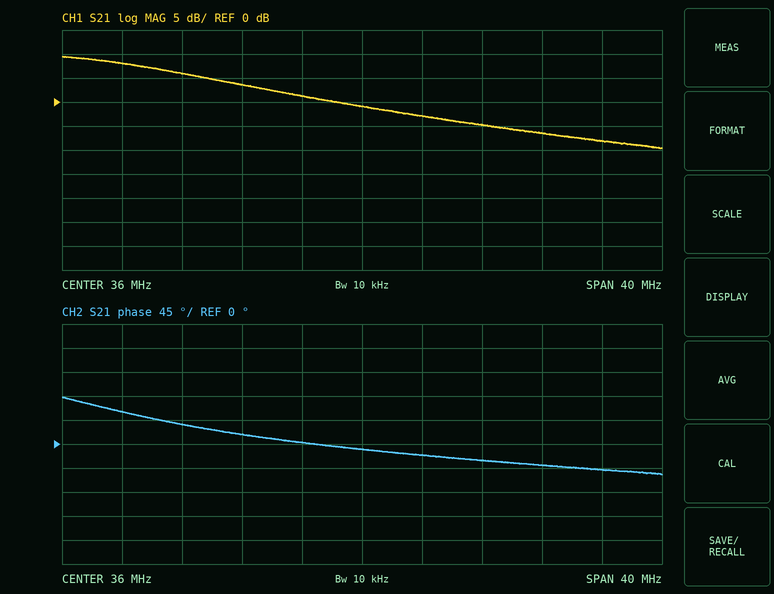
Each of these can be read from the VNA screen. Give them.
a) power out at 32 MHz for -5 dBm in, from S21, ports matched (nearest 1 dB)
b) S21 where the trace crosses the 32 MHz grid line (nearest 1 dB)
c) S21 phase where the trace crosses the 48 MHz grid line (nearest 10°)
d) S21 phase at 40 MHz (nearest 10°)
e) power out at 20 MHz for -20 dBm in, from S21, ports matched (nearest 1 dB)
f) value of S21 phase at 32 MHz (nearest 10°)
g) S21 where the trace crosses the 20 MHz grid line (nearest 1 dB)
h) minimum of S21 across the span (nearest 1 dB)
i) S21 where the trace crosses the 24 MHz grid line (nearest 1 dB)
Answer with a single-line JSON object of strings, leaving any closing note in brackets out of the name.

{"power out at 32 MHz for -5 dBm in, from S21, ports matched": "-4 dBm", "S21 where the trace crosses the 32 MHz grid line": "1 dB", "S21 phase where the trace crosses the 48 MHz grid line": "-40°", "S21 phase at 40 MHz": "-20°", "power out at 20 MHz for -20 dBm in, from S21, ports matched": "-12 dBm", "value of S21 phase at 32 MHz": "0°", "S21 where the trace crosses the 20 MHz grid line": "8 dB", "minimum of S21 across the span": "-10 dB", "S21 where the trace crosses the 24 MHz grid line": "6 dB"}
